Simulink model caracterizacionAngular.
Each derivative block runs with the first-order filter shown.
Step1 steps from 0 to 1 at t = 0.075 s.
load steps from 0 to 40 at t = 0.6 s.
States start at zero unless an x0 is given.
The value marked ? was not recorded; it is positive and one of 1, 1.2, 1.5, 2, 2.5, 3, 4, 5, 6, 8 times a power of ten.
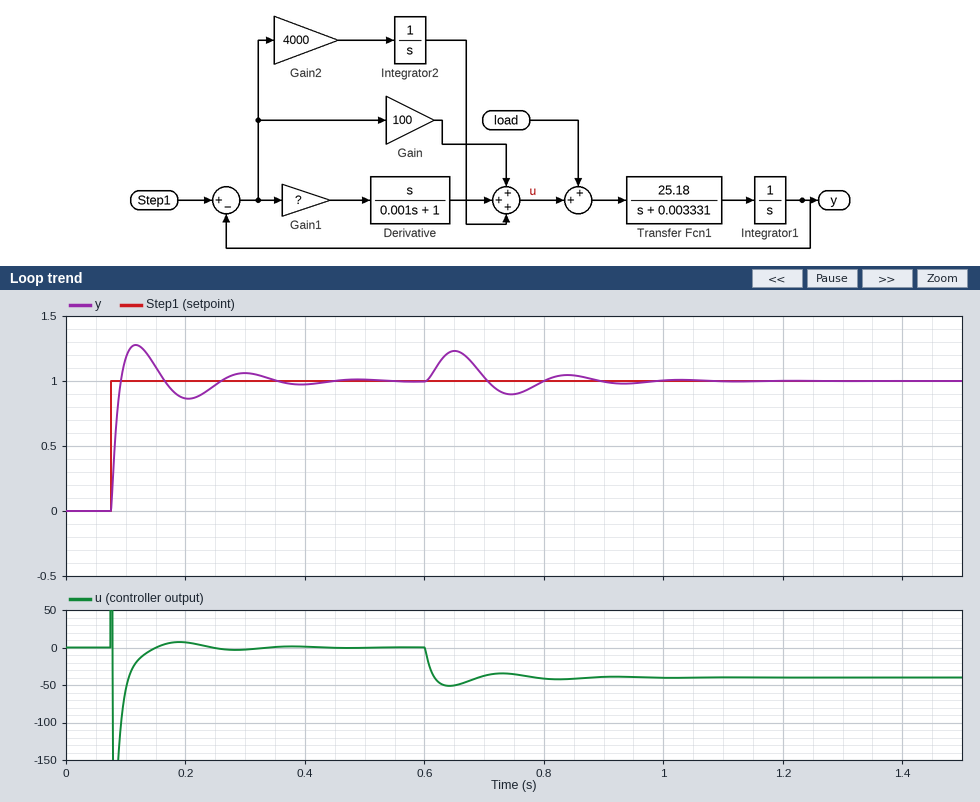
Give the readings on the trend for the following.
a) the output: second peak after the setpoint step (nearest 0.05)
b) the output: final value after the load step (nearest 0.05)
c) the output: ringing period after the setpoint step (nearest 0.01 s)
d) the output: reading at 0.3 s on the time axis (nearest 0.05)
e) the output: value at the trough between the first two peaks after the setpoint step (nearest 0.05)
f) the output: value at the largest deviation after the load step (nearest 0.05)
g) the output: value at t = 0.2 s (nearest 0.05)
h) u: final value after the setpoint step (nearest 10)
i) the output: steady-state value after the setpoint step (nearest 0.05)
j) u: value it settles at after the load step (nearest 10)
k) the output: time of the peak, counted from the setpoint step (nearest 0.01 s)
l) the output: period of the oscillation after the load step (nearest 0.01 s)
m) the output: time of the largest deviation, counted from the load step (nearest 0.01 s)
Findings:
1.05
1.00
0.18 s
1.05
0.85
1.25
0.85
0
1.00
-40
0.04 s
0.19 s
0.05 s
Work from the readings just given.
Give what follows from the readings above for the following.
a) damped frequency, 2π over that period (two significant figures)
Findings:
35 rad/s
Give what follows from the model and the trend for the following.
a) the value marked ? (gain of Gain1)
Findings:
4
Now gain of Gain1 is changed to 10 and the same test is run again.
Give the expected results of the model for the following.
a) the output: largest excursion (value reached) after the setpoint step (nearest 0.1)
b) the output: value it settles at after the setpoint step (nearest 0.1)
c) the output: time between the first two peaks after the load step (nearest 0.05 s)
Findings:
1.1
1.0
0.30 s
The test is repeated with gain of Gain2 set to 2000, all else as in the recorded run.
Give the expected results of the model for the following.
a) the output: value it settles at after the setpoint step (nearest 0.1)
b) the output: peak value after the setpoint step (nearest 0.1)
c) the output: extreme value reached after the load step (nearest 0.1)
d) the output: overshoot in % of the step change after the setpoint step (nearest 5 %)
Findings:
1.0
1.2
1.3
20 %
